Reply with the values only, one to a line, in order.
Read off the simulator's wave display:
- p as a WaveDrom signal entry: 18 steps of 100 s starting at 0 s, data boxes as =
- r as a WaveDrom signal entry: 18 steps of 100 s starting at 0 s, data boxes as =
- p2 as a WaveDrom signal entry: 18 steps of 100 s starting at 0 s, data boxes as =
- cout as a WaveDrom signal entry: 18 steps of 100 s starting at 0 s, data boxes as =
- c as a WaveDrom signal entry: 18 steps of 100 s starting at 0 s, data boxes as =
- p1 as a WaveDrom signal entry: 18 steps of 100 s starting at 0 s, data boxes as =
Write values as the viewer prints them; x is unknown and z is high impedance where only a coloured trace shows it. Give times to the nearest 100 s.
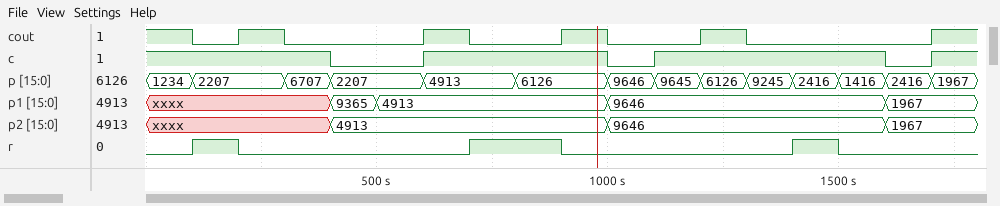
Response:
{name: 'p', wave: '==.==.=.=.========', data: '1234 2207 6707 2207 4913 6126 9646 9645 6126 9245 2416 1416 2416 1967'}
{name: 'r', wave: '010....1.0....10..'}
{name: 'p2', wave: 'x...=.....=.....=.', data: '4913 9646 1967'}
{name: 'cout', wave: '1010..10.10.10...1'}
{name: 'c', wave: '1...0.1...01....01'}
{name: 'p1', wave: 'x...==....=.....=.', data: '9365 4913 9646 1967'}
